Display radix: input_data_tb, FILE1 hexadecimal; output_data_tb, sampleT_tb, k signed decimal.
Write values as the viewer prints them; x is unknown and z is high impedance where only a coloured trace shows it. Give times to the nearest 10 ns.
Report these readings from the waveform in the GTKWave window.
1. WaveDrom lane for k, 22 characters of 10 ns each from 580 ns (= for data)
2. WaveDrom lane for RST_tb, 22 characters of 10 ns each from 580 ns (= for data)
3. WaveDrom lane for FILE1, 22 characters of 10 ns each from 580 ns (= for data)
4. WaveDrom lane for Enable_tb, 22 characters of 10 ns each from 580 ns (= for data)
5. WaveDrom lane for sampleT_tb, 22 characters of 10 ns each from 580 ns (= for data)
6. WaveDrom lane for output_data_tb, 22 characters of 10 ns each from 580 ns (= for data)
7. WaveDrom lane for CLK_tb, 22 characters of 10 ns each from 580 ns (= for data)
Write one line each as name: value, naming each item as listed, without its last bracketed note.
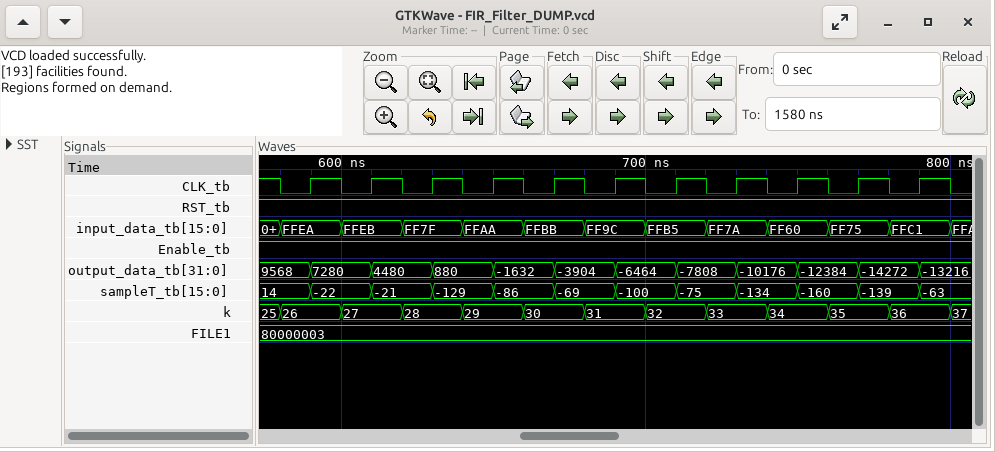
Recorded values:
WaveDrom lane for k, 22 characters of 10 ns each from 580 ns: {name: 'k', wave: '=.=.=.=.=.=.=.=.=.=.=.', data: '26 27 28 29 30 31 32 33 34 35 36'}
WaveDrom lane for RST_tb, 22 characters of 10 ns each from 580 ns: {name: 'RST_tb', wave: '1.....................'}
WaveDrom lane for FILE1, 22 characters of 10 ns each from 580 ns: {name: 'FILE1', wave: '=.....................', data: '80000003'}
WaveDrom lane for Enable_tb, 22 characters of 10 ns each from 580 ns: {name: 'Enable_tb', wave: '1.....................'}
WaveDrom lane for sampleT_tb, 22 characters of 10 ns each from 580 ns: {name: 'sampleT_tb', wave: '==.=.=.=.=.=.=.=.=.=.=', data: '14 -22 -21 -129 -86 -69 -100 -75 -134 -160 -139 -63'}
WaveDrom lane for output_data_tb, 22 characters of 10 ns each from 580 ns: {name: 'output_data_tb', wave: '==.=.=.=.=.=.=.=.=.=.=', data: '9568 7280 4480 880 -1632 -3904 -6464 -7808 -10176 -12384 -14272 -13216'}
WaveDrom lane for CLK_tb, 22 characters of 10 ns each from 580 ns: {name: 'CLK_tb', wave: '0101010101010101010101'}
